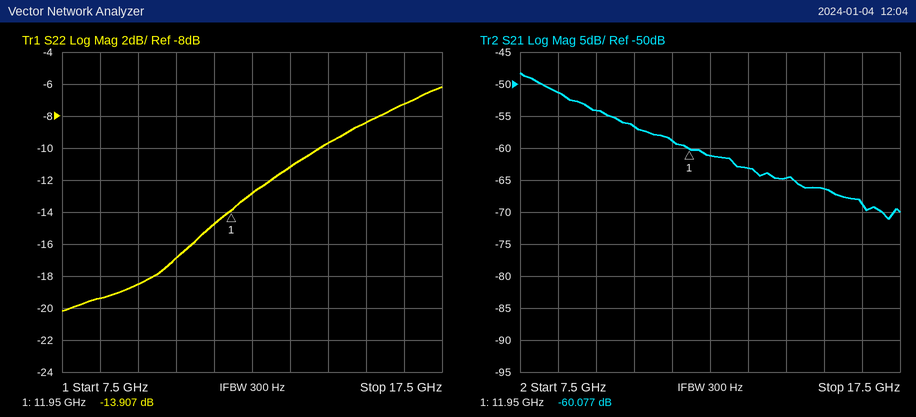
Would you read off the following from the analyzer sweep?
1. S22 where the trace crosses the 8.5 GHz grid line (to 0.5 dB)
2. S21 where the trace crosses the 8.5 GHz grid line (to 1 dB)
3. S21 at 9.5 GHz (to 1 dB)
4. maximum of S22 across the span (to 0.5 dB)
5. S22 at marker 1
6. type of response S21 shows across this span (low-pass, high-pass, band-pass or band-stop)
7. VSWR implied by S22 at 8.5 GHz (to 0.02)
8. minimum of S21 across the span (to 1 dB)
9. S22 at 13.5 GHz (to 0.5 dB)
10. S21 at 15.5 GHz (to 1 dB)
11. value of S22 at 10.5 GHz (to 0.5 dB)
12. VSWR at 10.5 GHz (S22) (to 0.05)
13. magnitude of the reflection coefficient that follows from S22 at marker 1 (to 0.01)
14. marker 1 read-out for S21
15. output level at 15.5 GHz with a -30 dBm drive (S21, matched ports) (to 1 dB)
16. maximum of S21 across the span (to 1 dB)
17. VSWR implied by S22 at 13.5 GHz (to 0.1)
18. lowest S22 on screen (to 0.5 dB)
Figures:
-19.5 dB
-51 dB
-54 dB
-6.0 dB
-13.907 dB
low-pass
1.24
-71 dB
-11.0 dB
-66 dB
-17.0 dB
1.35
0.20
-60.077 dB
-96 dBm
-48 dB
1.8
-20.0 dB
